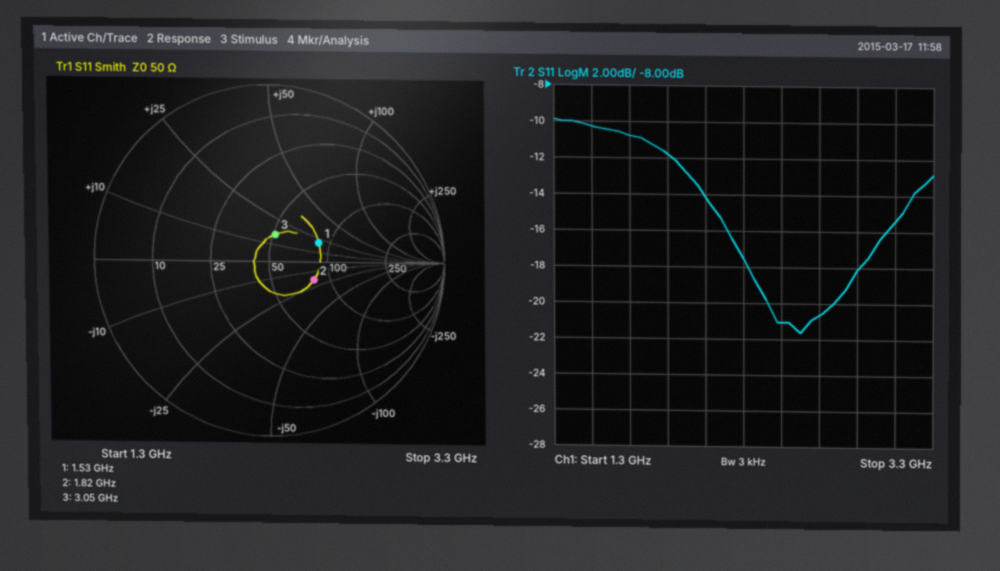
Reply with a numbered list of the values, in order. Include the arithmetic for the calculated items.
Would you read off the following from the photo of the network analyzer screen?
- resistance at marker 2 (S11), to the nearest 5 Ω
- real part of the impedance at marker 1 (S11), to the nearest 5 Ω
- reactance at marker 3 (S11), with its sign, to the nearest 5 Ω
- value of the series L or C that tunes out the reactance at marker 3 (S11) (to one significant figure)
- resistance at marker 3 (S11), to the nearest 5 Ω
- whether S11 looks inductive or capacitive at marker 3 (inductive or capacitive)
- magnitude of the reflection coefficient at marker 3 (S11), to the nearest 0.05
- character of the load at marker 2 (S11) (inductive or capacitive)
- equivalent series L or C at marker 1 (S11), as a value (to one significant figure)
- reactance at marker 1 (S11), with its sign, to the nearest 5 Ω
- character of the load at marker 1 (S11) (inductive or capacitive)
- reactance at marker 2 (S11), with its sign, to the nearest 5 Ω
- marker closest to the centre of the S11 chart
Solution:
1. 80 Ω
2. 85 Ω
3. +15 Ω
4. C = 1/(2π × 3.05 GHz × 15 Ω) ≈ 3 pF
5. 50 Ω
6. inductive
7. 0.15
8. capacitive
9. L = 20 Ω/(2π × 1.53 GHz) ≈ 2 nH
10. +20 Ω
11. inductive
12. -20 Ω
13. marker 3
